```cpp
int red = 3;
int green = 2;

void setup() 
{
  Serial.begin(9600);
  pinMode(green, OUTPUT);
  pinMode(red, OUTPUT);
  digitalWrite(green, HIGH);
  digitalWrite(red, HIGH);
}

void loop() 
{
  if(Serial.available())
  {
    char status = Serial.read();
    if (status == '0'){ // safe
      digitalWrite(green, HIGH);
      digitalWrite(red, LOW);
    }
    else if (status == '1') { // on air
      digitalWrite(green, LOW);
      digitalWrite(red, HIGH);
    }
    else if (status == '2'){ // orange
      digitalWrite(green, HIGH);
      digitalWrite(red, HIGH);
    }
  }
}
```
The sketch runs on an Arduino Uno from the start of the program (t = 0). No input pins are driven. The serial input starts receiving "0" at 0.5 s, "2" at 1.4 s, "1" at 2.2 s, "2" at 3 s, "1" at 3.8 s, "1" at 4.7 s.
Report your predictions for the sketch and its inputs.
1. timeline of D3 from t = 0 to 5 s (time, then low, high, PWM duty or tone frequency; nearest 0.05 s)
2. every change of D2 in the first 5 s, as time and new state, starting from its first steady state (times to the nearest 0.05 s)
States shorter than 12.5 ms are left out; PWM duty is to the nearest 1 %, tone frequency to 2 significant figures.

0 s high; 0.5 s low; 1.4 s high
0 s high; 2.2 s low; 3 s high; 3.8 s low
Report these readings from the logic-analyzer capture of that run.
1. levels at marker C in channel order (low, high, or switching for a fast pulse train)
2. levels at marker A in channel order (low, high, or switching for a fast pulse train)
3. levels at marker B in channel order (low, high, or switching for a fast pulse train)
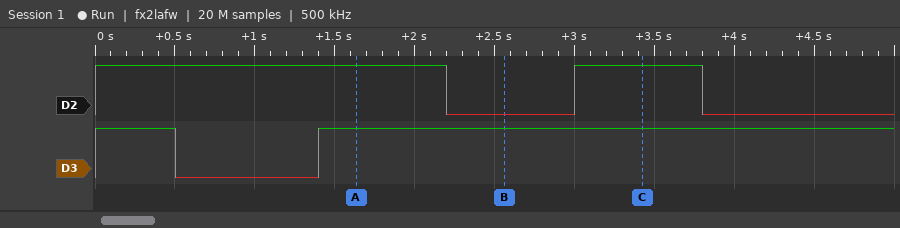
D2 high, D3 high
D2 high, D3 high
D2 low, D3 high
